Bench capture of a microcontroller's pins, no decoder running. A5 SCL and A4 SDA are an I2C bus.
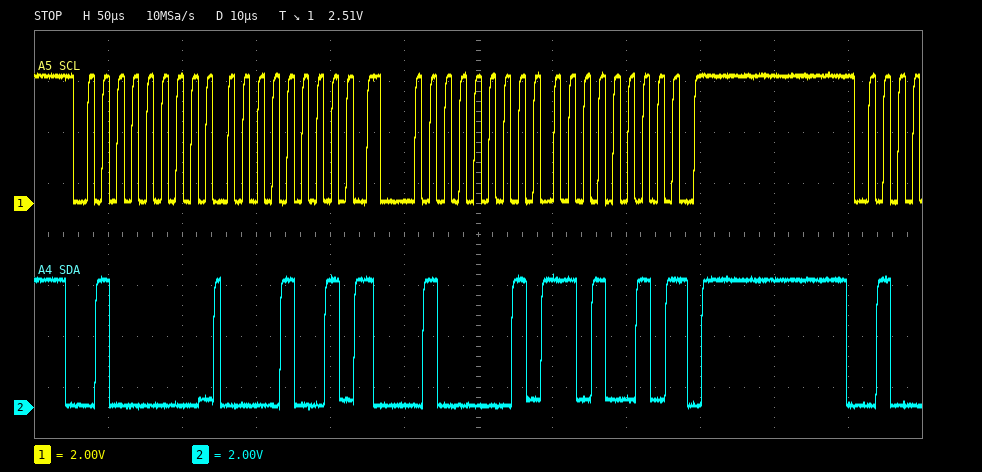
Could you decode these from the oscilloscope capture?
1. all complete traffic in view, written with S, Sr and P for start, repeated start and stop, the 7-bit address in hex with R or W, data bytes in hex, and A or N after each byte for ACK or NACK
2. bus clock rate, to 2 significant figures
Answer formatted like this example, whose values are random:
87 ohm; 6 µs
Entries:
S 20W A 09 A Sr 20R A D2 N P; 100 kHz
